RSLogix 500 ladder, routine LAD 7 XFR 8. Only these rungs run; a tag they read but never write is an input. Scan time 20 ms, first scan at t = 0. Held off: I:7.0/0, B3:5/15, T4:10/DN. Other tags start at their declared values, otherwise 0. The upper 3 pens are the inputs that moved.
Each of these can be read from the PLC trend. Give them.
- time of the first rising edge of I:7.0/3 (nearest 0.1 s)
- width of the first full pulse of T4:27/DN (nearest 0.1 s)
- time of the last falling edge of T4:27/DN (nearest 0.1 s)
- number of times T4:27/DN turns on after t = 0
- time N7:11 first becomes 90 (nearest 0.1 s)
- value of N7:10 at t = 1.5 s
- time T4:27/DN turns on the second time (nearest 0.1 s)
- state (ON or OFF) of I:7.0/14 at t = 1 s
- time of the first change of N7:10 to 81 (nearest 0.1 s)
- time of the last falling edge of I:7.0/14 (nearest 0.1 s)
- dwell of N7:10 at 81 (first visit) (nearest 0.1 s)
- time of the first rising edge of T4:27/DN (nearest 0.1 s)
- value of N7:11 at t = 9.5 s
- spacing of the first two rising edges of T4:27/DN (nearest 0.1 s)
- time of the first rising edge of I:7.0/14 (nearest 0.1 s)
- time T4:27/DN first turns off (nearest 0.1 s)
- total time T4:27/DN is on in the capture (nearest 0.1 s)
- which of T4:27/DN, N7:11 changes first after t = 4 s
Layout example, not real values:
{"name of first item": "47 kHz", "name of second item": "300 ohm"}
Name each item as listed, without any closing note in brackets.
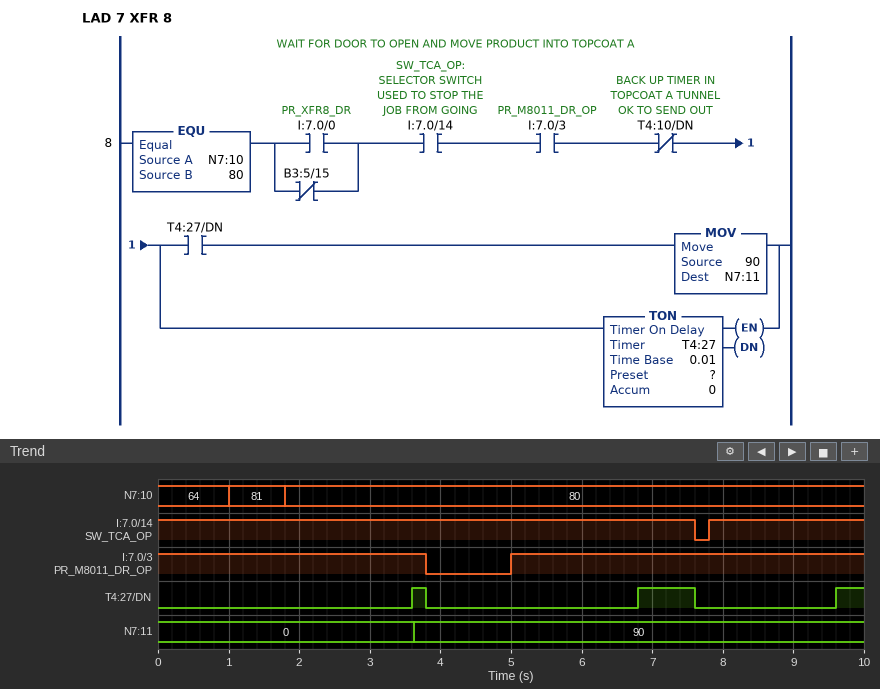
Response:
{"time of the first rising edge of I:7.0/3": "5.0 s", "width of the first full pulse of T4:27/DN": "0.2 s", "time of the last falling edge of T4:27/DN": "7.6 s", "number of times T4:27/DN turns on after t = 0": "3", "time N7:11 first becomes 90": "3.6 s", "value of N7:10 at t = 1.5 s": "81", "time T4:27/DN turns on the second time": "6.8 s", "state (ON or OFF) of I:7.0/14 at t = 1 s": "ON", "time of the first change of N7:10 to 81": "1.0 s", "time of the last falling edge of I:7.0/14": "7.6 s", "dwell of N7:10 at 81 (first visit)": "0.8 s", "time of the first rising edge of T4:27/DN": "3.6 s", "value of N7:11 at t = 9.5 s": "90", "spacing of the first two rising edges of T4:27/DN": "3.2 s", "time of the first rising edge of I:7.0/14": "7.8 s", "time T4:27/DN first turns off": "3.8 s", "total time T4:27/DN is on in the capture": "1.4 s", "which of T4:27/DN, N7:11 changes first after t = 4 s": "T4:27/DN"}
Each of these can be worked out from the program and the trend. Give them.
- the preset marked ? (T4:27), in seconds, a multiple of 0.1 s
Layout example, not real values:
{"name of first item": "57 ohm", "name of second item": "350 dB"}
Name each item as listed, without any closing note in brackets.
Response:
{"the preset marked ? (T4:27), in seconds, a multiple of 0.1 s": "1.8 s"}
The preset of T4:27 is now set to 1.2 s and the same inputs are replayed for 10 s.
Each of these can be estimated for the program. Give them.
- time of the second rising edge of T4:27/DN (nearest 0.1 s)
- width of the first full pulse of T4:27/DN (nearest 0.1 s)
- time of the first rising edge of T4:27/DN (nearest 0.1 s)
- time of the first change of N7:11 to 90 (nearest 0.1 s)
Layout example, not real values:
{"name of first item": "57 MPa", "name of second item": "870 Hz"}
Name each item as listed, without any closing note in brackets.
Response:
{"time of the second rising edge of T4:27/DN": "6.2 s", "width of the first full pulse of T4:27/DN": "0.8 s", "time of the first rising edge of T4:27/DN": "3.0 s", "time of the first change of N7:11 to 90": "3.0 s"}
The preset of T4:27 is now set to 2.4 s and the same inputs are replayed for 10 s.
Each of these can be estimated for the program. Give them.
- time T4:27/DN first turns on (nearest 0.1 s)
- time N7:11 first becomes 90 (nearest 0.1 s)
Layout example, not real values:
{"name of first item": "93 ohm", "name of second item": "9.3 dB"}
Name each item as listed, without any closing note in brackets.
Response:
{"time T4:27/DN first turns on": "7.4 s", "time N7:11 first becomes 90": "7.4 s"}
